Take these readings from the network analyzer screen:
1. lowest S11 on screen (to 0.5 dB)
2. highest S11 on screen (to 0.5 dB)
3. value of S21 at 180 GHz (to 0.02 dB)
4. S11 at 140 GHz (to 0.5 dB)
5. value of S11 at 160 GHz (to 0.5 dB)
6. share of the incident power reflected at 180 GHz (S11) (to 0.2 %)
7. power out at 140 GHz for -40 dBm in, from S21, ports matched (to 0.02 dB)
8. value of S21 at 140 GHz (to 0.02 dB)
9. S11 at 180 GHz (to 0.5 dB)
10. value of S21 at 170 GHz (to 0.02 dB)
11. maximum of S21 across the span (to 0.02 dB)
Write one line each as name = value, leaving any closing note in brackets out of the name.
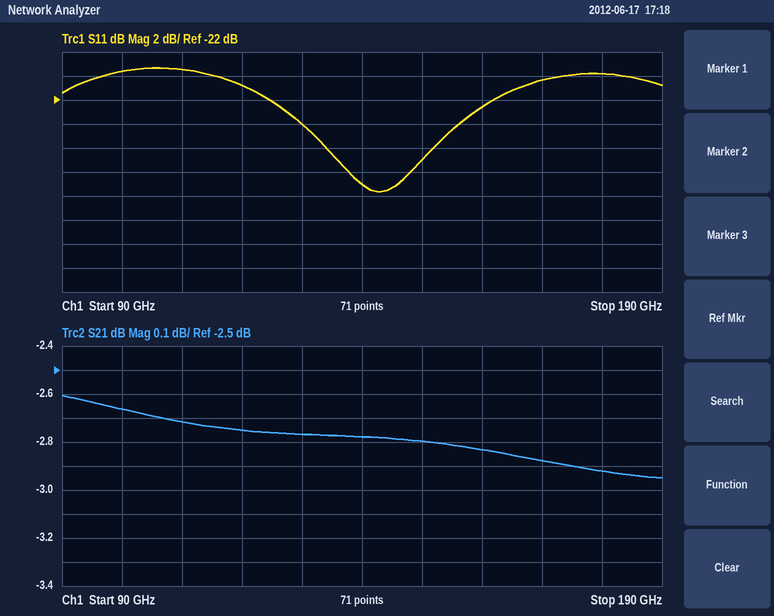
lowest S11 on screen = -29.5 dB
highest S11 on screen = -19.5 dB
value of S21 at 180 GHz = -2.92 dB
S11 at 140 GHz = -29.0 dB
value of S11 at 160 GHz = -22.5 dB
share of the incident power reflected at 180 GHz (S11) = 1.0 %
power out at 140 GHz for -40 dBm in, from S21, ports matched = -42.78 dBm
value of S21 at 140 GHz = -2.78 dB
S11 at 180 GHz = -20.0 dB
value of S21 at 170 GHz = -2.88 dB
maximum of S21 across the span = -2.60 dB
